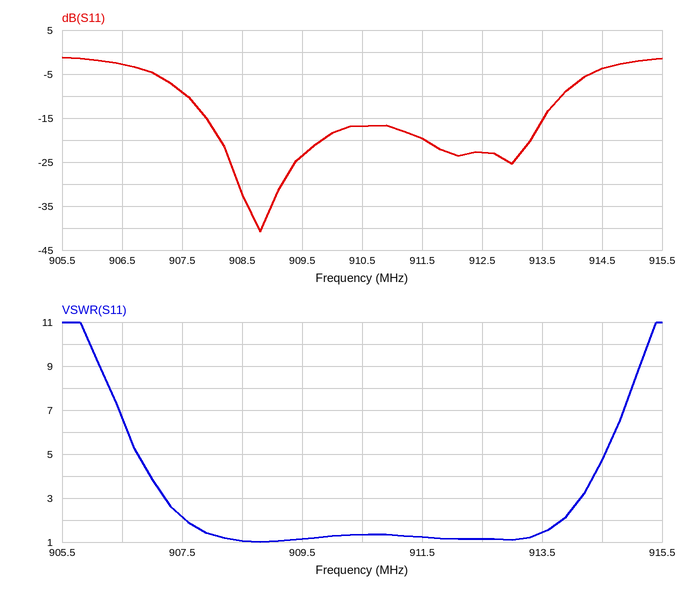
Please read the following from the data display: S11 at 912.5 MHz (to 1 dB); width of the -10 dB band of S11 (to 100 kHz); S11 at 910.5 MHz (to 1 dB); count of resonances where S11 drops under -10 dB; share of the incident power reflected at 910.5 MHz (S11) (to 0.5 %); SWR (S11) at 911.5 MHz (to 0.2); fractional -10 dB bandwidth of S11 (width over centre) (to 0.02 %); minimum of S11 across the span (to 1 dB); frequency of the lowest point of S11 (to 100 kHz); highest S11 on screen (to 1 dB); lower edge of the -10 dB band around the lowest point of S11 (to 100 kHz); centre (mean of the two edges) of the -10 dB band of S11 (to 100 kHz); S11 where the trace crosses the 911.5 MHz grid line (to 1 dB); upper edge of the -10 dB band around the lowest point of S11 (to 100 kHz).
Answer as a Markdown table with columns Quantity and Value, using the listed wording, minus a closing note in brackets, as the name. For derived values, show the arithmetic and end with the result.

| Quantity | Value |
|---|---|
| S11 at 912.5 MHz | -23 dB |
| width of the -10 dB band of S11 | 913.8 MHz − 907.6 MHz = 6.2 MHz |
| S11 at 910.5 MHz | -17 dB |
| count of resonances where S11 drops under -10 dB | 2 |
| share of the incident power reflected at 910.5 MHz (S11) | 10^(-17/10) ≈ 2.0 % |
| SWR (S11) at 911.5 MHz | 1.2 |
| fractional -10 dB bandwidth of S11 (width over centre) | 6.2 MHz / 910.7 MHz ≈ 0.68 % |
| minimum of S11 across the span | -41 dB |
| frequency of the lowest point of S11 | 908.8 MHz |
| highest S11 on screen | -1 dB |
| lower edge of the -10 dB band around the lowest point of S11 | 907.6 MHz |
| centre (mean of the two edges) of the -10 dB band of S11 | 910.7 MHz |
| S11 where the trace crosses the 911.5 MHz grid line | -20 dB |
| upper edge of the -10 dB band around the lowest point of S11 | 913.8 MHz |
